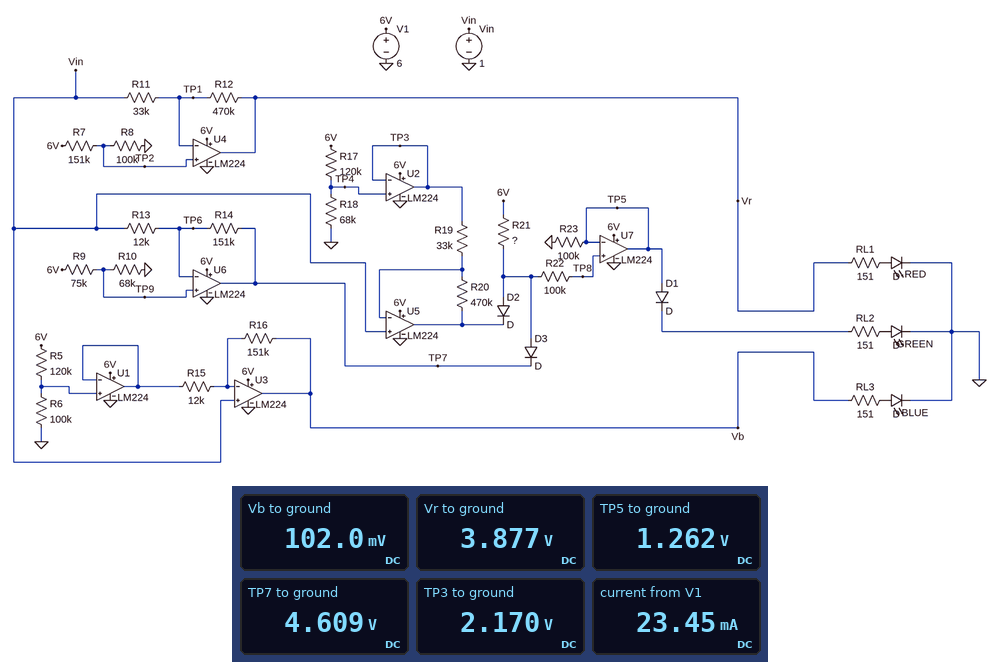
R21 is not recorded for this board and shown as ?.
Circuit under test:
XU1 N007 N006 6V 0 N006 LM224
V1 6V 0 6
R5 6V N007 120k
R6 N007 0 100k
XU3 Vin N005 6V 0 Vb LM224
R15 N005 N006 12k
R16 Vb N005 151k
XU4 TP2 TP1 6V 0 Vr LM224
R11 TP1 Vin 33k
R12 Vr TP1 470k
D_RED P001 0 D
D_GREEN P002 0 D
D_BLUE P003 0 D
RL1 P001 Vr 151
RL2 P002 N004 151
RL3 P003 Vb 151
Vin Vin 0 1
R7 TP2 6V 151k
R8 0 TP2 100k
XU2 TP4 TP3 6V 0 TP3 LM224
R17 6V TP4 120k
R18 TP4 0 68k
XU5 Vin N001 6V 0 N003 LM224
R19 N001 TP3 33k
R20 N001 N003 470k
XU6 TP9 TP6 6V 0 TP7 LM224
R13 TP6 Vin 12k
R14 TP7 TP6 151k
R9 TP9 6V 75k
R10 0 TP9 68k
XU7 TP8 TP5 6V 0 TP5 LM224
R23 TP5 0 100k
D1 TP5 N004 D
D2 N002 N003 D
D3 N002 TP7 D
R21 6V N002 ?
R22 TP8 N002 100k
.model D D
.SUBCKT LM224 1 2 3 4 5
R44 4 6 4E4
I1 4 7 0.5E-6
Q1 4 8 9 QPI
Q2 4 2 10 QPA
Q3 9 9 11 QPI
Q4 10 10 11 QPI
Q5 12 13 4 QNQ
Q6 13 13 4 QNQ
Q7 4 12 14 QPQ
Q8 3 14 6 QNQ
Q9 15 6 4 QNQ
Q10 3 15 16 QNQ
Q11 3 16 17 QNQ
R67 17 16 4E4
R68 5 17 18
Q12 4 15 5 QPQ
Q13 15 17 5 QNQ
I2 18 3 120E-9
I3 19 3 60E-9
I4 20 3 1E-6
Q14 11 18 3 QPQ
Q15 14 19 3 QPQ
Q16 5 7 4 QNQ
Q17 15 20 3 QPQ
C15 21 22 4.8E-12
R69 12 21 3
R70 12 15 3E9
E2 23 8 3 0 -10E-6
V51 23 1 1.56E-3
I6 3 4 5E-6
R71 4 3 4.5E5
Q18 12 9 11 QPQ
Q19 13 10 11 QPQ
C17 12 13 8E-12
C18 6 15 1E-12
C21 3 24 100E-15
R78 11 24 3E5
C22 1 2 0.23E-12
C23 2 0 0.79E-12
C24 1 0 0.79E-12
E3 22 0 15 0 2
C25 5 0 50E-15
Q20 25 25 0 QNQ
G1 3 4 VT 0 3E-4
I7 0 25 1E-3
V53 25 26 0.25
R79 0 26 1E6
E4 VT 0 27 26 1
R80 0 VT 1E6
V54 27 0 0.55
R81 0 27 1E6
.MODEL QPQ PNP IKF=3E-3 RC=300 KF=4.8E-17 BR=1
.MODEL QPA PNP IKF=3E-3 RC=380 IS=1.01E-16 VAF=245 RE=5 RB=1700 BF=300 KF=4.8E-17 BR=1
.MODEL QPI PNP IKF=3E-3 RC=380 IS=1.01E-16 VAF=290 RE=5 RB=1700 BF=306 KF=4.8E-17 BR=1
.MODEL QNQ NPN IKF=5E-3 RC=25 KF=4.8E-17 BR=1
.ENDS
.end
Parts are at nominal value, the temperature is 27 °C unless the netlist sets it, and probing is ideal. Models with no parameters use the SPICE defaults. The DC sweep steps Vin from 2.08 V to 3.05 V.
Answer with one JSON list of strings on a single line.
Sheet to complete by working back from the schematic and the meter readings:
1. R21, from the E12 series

["68 kΩ"]
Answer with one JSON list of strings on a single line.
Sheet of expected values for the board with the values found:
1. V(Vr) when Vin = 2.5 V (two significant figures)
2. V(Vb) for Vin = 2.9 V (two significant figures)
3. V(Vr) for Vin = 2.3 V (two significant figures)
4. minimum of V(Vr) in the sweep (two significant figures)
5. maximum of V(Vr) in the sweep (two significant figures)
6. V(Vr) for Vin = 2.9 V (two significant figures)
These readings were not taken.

["830 mV", "3.9 V", "3.7 V", "67 mV", "3.9 V", "70 mV"]
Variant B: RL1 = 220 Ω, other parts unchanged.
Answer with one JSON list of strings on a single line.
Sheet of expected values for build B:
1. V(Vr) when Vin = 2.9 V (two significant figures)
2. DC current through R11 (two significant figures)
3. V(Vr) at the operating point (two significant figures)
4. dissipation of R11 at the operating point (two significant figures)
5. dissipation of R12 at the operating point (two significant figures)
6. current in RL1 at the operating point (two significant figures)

["70 mV", "6.0 µA", "4.0 V", "1.2 µW", "17 µW", "15 mA"]
